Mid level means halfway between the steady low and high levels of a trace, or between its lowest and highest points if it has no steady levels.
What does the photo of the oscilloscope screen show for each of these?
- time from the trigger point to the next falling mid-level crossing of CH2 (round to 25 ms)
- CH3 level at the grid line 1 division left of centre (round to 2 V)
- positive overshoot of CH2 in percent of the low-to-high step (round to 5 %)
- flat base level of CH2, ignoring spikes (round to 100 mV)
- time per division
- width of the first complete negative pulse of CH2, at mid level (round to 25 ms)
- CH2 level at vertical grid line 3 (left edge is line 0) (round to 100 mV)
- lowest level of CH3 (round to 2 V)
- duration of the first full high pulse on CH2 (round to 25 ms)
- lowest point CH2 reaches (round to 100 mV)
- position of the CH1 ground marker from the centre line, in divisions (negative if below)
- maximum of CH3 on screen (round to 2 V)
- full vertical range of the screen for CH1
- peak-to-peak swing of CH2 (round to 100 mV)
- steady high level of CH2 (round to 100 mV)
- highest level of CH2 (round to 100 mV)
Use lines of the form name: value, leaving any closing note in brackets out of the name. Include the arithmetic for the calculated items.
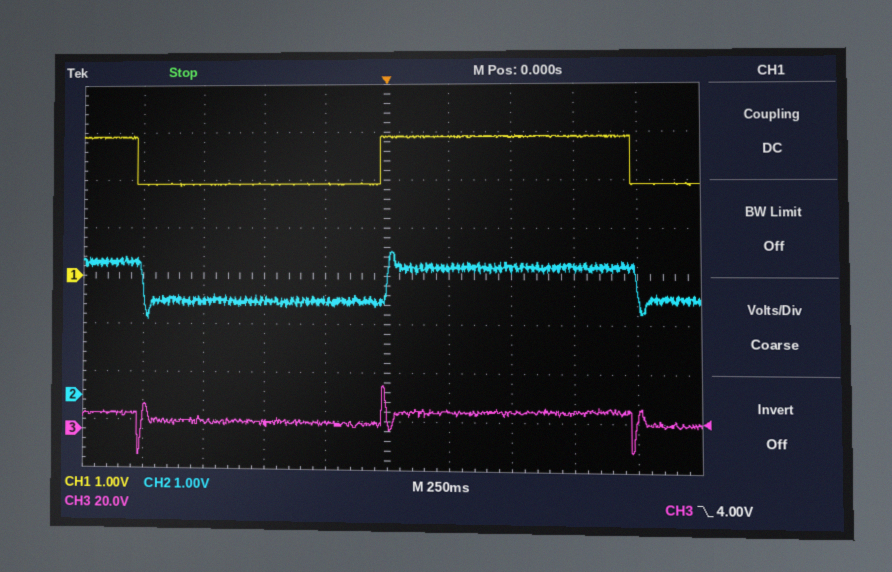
time from the trigger point to the next falling mid-level crossing of CH2: 1.000 s
CH3 level at the grid line 1 division left of centre: 4 V
positive overshoot of CH2 in percent of the low-to-high step: 45 %
flat base level of CH2, ignoring spikes: 2.0 V
time per division: 250 ms
width of the first complete negative pulse of CH2, at mid level: 1.000 s
CH2 level at vertical grid line 3 (left edge is line 0): 2.0 V
lowest level of CH3: -10 V
duration of the first full high pulse on CH2: 1.000 s
lowest point CH2 reaches: 1.6 V
position of the CH1 ground marker from the centre line, in divisions: 0.0 div
maximum of CH3 on screen: 18 V
full vertical range of the screen for CH1: 8 V
peak-to-peak swing of CH2: 3.0 V − (1.6 V) = 1.4 V
steady high level of CH2: 2.7 V
highest level of CH2: 3.0 V
